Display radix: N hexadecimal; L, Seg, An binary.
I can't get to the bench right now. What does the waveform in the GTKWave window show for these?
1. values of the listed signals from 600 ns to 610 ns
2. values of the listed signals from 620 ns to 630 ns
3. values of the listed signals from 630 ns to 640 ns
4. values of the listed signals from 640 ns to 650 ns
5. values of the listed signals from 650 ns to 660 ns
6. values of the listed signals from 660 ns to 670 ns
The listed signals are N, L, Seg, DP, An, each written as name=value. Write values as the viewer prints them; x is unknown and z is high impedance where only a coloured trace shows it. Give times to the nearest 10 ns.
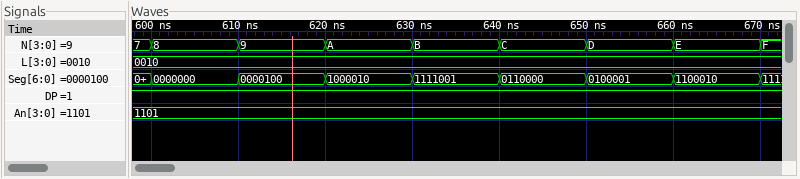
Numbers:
N=8, L=0010, Seg=0000000, DP=1, An=1101
N=A, L=0010, Seg=1000010, DP=1, An=1101
N=B, L=0010, Seg=1111001, DP=1, An=1101
N=C, L=0010, Seg=0110000, DP=1, An=1101
N=D, L=0010, Seg=0100001, DP=1, An=1101
N=E, L=0010, Seg=1100010, DP=1, An=1101
